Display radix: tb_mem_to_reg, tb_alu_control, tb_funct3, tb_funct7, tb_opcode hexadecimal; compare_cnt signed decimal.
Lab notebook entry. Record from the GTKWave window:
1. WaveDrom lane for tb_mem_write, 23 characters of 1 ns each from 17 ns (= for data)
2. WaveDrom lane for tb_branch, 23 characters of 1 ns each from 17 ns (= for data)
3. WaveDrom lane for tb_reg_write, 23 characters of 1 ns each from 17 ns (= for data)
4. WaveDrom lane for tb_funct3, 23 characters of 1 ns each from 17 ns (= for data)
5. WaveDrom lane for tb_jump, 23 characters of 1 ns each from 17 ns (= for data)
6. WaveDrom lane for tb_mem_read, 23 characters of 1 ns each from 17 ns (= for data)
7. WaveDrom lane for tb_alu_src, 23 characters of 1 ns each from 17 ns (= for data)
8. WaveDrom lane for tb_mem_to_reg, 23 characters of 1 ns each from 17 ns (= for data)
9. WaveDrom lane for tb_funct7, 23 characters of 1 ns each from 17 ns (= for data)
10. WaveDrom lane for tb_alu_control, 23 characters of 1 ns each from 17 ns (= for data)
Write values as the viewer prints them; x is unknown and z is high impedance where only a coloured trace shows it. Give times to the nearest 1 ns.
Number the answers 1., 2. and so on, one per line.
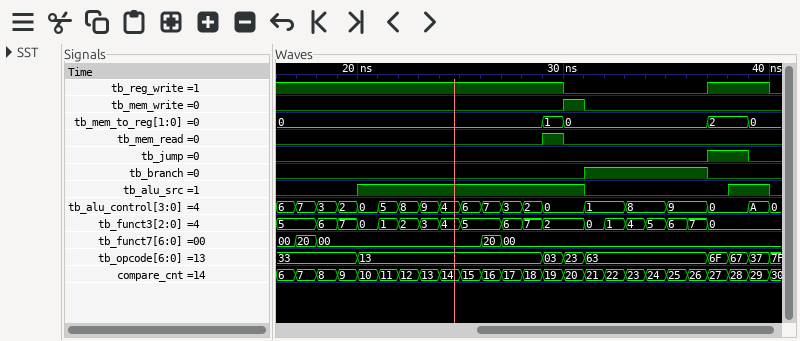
1. {name: 'tb_mem_write', wave: '0............10........'}
2. {name: 'tb_branch', wave: '0.............1.....0..'}
3. {name: 'tb_reg_write', wave: '1............0......1..'}
4. {name: 'tb_funct3', wave: '=========.===.=======..', data: '5 6 7 0 1 2 3 4 5 6 7 2 0 1 4 5 6 7 0'}
5. {name: 'tb_jump', wave: '0...................1.0'}
6. {name: 'tb_mem_read', wave: '0...........10.........'}
7. {name: 'tb_alu_src', wave: '0..1..........0......1.'}
8. {name: 'tb_mem_to_reg', wave: '=...........==......=.=', data: '0 1 0 2 0'}
9. {name: 'tb_funct7', wave: '==.......==............', data: '20 00 20 00'}
10. {name: 'tb_alu_control', wave: '=============.=.=.=.=.=', data: '7 3 2 0 5 8 9 4 6 7 3 2 0 1 8 9 0 A'}
